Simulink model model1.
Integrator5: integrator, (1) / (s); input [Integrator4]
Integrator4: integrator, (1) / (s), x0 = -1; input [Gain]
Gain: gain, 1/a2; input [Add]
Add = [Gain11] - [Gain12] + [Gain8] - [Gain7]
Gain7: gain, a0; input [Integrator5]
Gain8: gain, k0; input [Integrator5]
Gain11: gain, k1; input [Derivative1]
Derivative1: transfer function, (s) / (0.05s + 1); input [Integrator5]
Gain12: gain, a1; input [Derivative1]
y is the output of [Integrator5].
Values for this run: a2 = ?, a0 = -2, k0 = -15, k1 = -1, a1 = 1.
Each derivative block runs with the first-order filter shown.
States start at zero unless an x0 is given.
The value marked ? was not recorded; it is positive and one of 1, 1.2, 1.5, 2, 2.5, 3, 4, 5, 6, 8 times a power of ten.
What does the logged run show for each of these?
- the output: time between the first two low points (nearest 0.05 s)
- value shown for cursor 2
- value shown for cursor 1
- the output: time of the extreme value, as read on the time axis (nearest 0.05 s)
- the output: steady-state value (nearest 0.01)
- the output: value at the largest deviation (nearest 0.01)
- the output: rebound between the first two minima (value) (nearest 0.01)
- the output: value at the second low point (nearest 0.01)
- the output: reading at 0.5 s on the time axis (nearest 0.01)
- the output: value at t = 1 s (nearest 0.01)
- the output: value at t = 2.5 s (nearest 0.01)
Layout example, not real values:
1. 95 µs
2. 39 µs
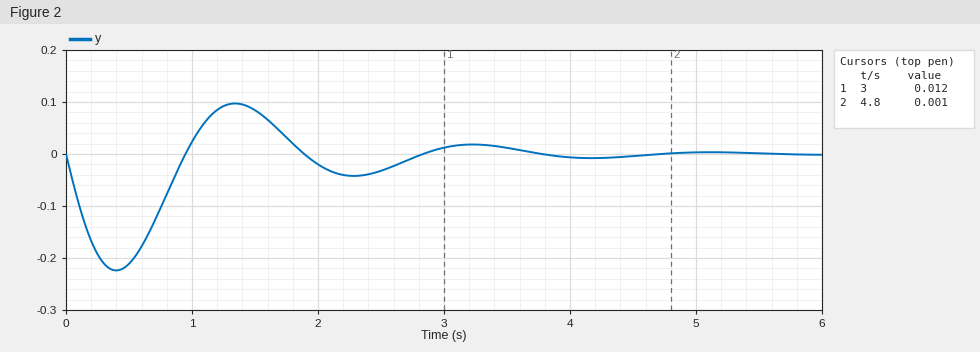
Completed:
1. 1.90 s
2. 0.001
3. 0.012
4. 0.40 s
5. 0.00
6. -0.22
7. 0.10
8. -0.04
9. -0.21
10. 0.02
11. -0.03
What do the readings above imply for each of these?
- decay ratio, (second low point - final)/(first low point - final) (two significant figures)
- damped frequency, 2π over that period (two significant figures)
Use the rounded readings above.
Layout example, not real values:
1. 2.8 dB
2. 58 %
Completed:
1. 0.18
2. 3.3 rad/s
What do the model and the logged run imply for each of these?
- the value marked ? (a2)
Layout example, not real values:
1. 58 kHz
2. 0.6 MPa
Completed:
1. 1.2
